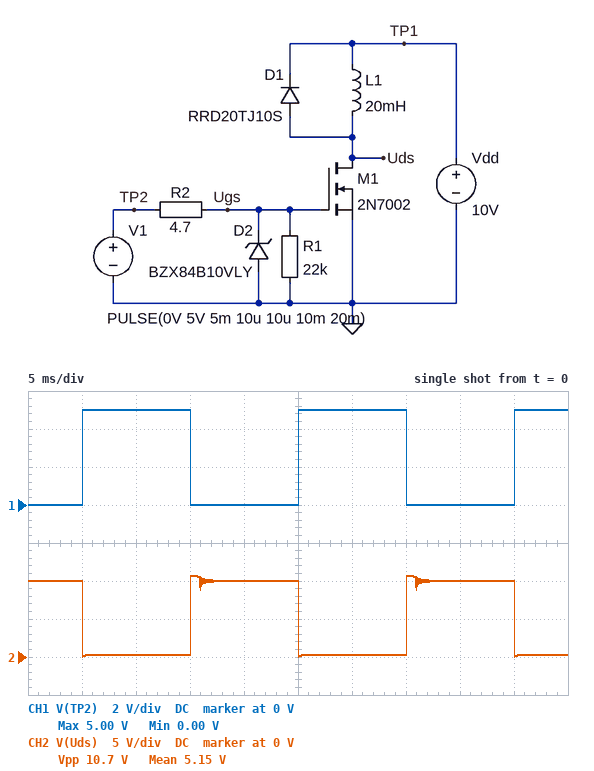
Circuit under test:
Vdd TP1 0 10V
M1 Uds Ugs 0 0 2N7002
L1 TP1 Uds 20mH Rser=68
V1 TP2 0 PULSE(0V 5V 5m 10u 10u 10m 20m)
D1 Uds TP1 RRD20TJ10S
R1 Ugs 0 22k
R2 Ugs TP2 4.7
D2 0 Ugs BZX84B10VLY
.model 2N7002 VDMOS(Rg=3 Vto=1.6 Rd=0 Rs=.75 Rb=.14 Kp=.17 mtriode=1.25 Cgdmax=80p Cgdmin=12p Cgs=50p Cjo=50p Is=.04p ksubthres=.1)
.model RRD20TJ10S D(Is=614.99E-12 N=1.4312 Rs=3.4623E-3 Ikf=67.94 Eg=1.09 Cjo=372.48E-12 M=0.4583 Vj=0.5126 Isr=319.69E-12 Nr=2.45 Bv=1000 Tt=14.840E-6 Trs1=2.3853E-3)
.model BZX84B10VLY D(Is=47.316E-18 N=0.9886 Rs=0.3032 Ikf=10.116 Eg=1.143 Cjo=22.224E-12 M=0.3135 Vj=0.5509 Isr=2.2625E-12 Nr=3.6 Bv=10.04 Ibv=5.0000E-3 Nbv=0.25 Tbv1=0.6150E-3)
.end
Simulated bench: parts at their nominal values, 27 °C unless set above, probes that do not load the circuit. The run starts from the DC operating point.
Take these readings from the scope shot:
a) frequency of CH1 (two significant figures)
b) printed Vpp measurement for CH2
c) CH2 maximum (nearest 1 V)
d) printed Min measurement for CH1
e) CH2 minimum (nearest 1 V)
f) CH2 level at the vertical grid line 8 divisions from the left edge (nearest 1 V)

50 Hz
10.7 V
11 V
0.00 V
0 V
10 V
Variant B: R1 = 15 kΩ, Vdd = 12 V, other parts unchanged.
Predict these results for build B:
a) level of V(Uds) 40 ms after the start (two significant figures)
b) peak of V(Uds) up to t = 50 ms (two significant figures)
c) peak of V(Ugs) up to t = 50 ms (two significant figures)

12 V
13 V
5.0 V
